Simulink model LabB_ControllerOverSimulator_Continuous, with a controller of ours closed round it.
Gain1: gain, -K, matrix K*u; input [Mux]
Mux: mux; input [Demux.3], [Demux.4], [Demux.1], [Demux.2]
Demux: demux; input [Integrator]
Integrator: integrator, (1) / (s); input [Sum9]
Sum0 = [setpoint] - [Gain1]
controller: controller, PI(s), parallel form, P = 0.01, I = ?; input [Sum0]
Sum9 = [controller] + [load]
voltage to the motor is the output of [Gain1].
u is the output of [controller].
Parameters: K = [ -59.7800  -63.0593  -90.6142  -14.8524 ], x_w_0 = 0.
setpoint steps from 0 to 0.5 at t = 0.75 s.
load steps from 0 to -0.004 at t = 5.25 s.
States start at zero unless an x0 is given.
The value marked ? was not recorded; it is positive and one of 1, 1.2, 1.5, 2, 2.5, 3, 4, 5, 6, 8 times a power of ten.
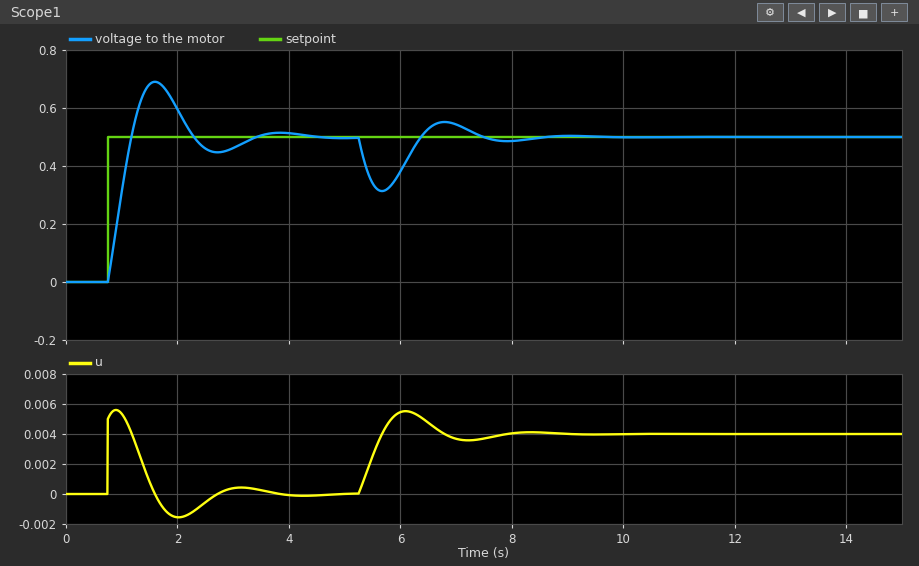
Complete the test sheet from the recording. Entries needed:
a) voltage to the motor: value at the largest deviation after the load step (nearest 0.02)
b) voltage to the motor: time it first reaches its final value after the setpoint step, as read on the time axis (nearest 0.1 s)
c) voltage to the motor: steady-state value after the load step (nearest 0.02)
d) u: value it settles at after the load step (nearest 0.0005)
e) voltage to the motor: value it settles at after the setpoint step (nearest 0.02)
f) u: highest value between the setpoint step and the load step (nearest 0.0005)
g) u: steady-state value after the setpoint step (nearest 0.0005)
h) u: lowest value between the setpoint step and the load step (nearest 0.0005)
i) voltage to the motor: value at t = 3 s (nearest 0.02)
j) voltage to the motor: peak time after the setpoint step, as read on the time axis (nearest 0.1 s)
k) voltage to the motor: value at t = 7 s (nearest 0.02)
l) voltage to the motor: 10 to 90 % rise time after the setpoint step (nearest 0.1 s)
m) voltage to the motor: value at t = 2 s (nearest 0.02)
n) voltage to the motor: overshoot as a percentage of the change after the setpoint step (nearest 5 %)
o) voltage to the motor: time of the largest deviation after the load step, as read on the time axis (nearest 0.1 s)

0.32
1.2 s
0.50
0.0040
0.50
0.0055
0.0000
-0.0015
0.46
1.6 s
0.54
0.3 s
0.60
40 %
5.7 s
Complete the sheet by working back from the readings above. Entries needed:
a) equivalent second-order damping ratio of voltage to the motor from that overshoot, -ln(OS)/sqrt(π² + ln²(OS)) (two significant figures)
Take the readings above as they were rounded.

0.28
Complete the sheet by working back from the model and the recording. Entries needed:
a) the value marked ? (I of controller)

0.04
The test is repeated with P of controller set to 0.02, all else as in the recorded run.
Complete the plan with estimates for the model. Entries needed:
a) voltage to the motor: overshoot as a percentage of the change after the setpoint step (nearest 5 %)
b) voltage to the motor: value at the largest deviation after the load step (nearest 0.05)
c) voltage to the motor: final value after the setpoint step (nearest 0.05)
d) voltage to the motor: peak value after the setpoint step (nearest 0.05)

20 %
0.35
0.50
0.60
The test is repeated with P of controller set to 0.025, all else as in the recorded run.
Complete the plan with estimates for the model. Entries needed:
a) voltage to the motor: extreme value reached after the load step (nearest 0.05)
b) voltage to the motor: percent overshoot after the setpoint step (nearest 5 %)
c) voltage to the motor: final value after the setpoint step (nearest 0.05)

0.40
15 %
0.50
